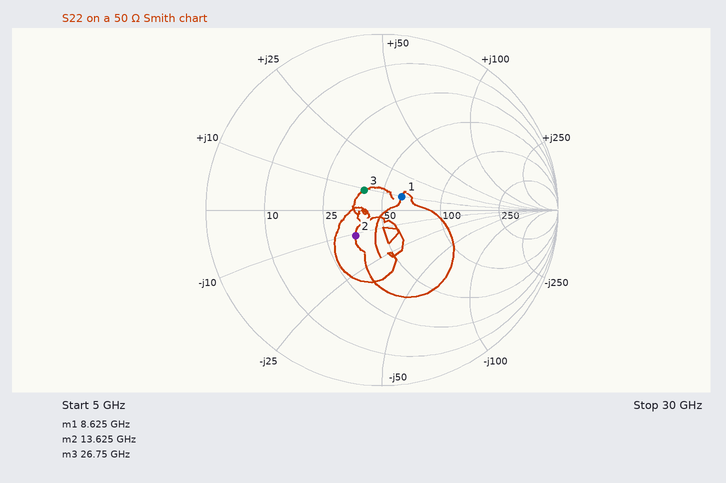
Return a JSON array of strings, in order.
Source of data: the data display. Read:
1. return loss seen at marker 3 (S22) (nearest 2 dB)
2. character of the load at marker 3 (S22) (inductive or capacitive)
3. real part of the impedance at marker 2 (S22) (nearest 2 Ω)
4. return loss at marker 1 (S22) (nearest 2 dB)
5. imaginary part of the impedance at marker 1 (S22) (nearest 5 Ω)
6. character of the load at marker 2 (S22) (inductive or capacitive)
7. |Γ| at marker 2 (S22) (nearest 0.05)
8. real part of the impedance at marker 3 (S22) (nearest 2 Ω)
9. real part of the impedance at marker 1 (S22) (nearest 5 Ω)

["16 dB", "inductive", "36 Ω", "18 dB", "+10 Ω", "capacitive", "0.20", "40 Ω", "60 Ω"]
